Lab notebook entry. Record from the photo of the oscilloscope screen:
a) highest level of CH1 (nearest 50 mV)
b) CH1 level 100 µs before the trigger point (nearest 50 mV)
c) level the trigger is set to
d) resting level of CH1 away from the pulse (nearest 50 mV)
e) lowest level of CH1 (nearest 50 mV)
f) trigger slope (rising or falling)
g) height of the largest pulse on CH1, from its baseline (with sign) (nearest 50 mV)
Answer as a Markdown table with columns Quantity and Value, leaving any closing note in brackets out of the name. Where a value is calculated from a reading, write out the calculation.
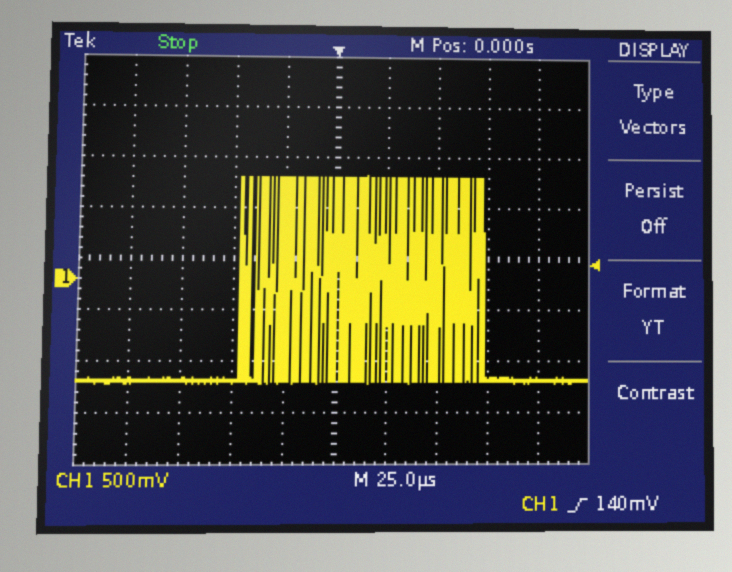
| Quantity | Value |
|---|---|
| highest level of CH1 | 1.00 V |
| CH1 level 100 µs before the trigger point | -1.00 V |
| level the trigger is set to | 140 mV |
| resting level of CH1 away from the pulse | -1.00 V |
| lowest level of CH1 | -1.00 V |
| trigger slope | rising |
| height of the largest pulse on CH1, from its baseline (with sign) | 1.00 V − (-1.00 V) = +2.00 V |
